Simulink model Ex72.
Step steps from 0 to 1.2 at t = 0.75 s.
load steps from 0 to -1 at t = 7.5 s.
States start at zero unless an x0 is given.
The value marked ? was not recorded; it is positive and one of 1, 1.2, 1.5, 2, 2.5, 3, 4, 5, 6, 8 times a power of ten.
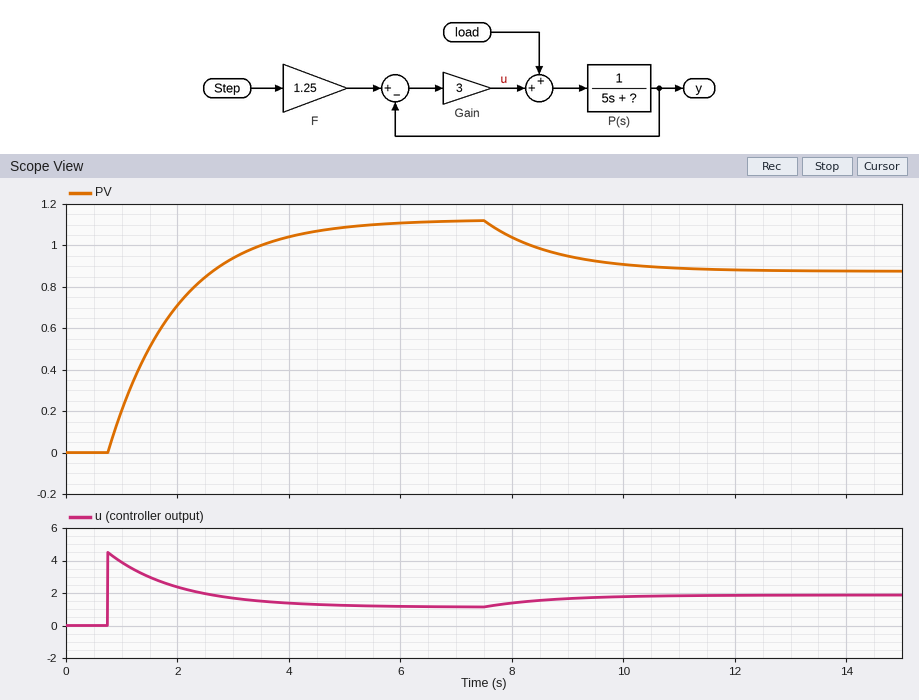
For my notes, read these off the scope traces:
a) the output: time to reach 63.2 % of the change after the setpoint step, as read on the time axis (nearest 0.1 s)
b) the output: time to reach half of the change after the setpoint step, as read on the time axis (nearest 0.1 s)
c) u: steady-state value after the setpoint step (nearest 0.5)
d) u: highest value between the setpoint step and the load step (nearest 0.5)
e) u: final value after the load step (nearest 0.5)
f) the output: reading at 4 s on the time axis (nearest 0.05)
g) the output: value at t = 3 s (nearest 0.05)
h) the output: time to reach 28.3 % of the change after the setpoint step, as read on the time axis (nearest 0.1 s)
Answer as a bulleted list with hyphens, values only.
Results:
- 2.0 s
- 1.6 s
- 1.0
- 4.5
- 2.0
- 1.05
- 0.95
- 1.2 s
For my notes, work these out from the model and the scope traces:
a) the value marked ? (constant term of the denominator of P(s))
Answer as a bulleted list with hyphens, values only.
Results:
- 1
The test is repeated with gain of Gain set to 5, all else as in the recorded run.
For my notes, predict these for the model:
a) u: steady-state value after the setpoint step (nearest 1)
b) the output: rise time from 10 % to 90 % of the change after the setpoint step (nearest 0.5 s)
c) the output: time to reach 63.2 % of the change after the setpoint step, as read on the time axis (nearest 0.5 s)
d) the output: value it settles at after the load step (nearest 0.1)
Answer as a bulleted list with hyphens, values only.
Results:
- 1
- 2.0 s
- 1.5 s
- 1.1
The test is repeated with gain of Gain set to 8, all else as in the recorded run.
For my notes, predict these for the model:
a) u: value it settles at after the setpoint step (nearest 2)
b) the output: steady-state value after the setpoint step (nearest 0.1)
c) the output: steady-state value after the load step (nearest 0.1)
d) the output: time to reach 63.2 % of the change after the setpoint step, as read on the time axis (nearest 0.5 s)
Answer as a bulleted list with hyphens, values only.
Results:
- 2
- 1.3
- 1.2
- 1.5 s
